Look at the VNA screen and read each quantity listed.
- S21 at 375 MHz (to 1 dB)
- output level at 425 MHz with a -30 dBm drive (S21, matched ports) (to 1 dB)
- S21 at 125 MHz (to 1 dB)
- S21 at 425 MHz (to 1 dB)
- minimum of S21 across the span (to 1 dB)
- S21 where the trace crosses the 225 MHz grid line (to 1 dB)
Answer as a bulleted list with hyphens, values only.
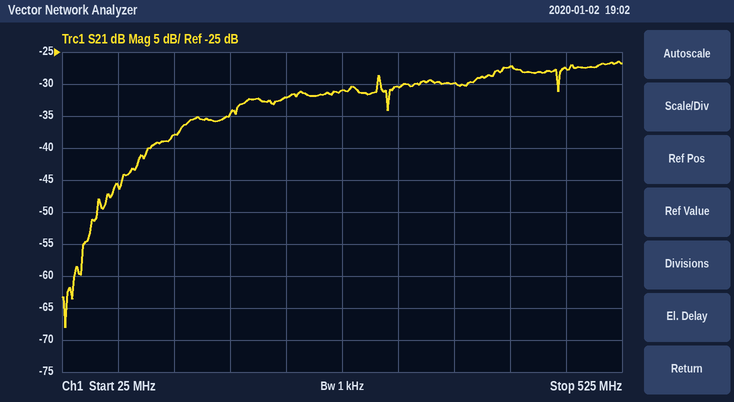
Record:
- -30 dB
- -57 dBm
- -38 dB
- -27 dB
- -68 dB
- -32 dB
